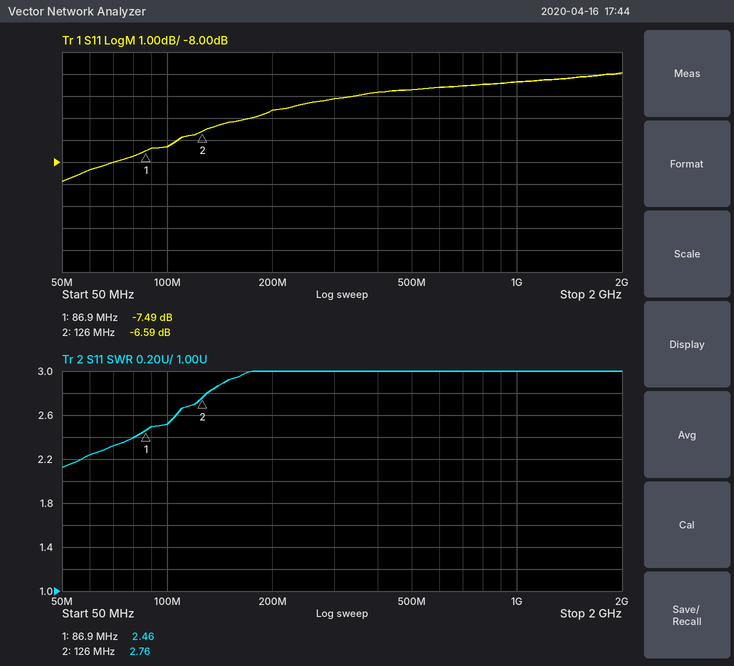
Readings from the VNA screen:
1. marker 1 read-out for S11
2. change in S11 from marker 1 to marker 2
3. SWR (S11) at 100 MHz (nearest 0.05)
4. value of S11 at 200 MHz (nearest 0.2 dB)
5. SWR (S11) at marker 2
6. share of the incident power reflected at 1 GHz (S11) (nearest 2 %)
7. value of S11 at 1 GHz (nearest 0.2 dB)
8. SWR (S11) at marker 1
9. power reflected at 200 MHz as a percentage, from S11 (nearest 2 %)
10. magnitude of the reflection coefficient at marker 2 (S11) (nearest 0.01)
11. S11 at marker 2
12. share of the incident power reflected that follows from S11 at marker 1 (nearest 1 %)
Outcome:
-7.49 dB
0.90 dB
2.50
-5.6 dB
2.76
36 %
-4.4 dB
2.46
28 %
0.47
-6.59 dB
18 %
